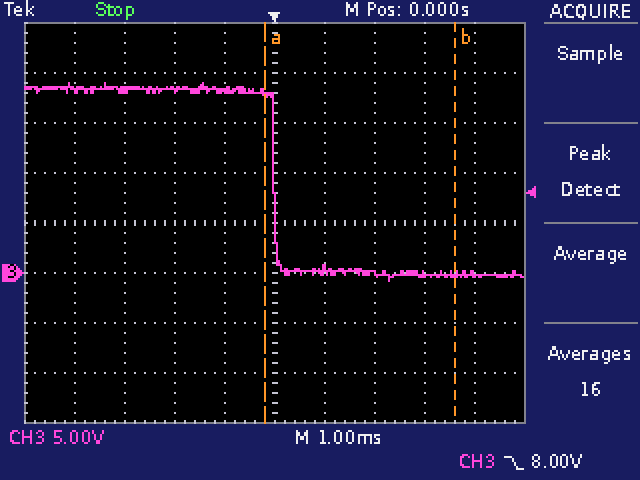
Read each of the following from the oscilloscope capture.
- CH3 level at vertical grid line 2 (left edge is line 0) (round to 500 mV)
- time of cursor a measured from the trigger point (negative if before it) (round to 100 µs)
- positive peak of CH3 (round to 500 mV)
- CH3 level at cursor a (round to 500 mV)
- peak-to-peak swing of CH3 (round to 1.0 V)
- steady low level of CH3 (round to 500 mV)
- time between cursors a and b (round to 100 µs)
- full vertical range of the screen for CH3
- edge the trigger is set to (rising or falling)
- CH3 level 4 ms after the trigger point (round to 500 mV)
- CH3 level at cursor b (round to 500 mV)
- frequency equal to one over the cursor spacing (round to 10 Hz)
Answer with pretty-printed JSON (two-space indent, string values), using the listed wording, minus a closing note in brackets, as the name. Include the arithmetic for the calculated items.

{
  "CH3 level at vertical grid line 2 (left edge is line 0)": "18.5 V",
  "time of cursor a measured from the trigger point (negative if before it)": "-200 µs",
  "positive peak of CH3": "19.0 V",
  "CH3 level at cursor a": "18.0 V",
  "peak-to-peak swing of CH3": "20.0 V",
  "steady low level of CH3": "0.0 V",
  "time between cursors a and b": "3.8 ms",
  "full vertical range of the screen for CH3": "40 V",
  "edge the trigger is set to": "falling",
  "CH3 level 4 ms after the trigger point": "0.0 V",
  "CH3 level at cursor b": "0.0 V",
  "frequency equal to one over the cursor spacing": "1 / 3.8 ms ≈ 260 Hz"
}
